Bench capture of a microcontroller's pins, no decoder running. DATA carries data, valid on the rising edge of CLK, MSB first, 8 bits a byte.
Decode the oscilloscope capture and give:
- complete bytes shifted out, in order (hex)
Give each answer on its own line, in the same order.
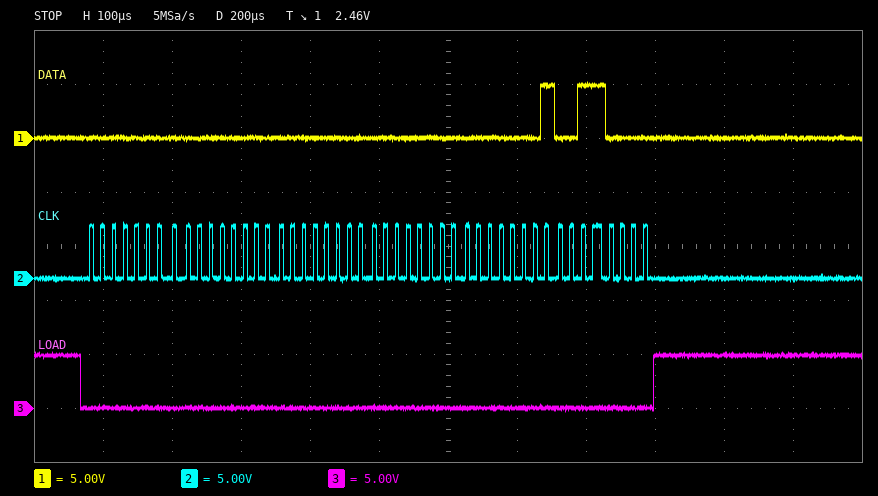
0x00 0x00 0x00 0x00 0x01 0x30
